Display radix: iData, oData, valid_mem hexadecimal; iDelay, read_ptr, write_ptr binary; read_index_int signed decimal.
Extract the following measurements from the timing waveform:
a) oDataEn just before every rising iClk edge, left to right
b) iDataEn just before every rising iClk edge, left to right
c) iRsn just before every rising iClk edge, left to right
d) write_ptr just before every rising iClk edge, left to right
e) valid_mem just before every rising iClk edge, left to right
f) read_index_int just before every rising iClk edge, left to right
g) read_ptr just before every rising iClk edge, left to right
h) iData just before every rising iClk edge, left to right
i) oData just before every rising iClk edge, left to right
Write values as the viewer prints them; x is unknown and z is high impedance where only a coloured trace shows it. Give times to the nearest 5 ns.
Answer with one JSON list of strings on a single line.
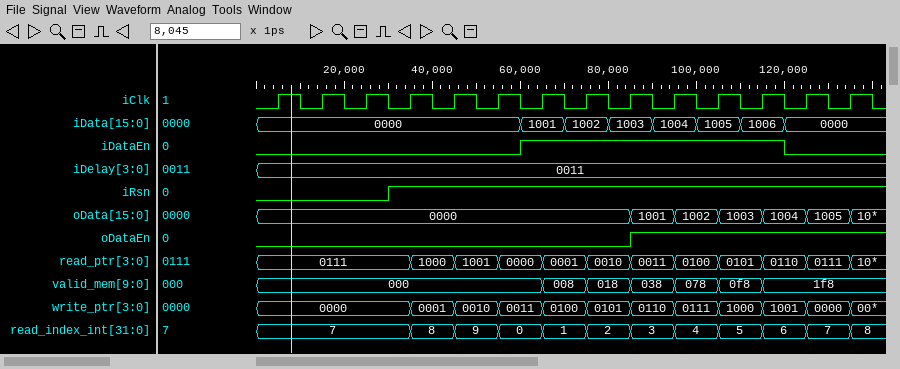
["0 0 0 0 0 0 0 0 0 1 1 1 1 1", "0 0 0 0 0 0 1 1 1 1 1 1 0 0", "0 0 0 1 1 1 1 1 1 1 1 1 1 1", "0000, 0000, 0000, 0000, 0001, 0010, 0011, 0100, 0101, 0110, 0111, 1000, 1001, 0000", "000, 000, 000, 000, 000, 000, 000, 008, 018, 038, 078, 0f8, 1f8, 1f8", "7, 7, 7, 7, 8, 9, 0, 1, 2, 3, 4, 5, 6, 7", "0111, 0111, 0111, 0111, 1000, 1001, 0000, 0001, 0010, 0011, 0100, 0101, 0110, 0111", "0000, 0000, 0000, 0000, 0000, 0000, 1001, 1002, 1003, 1004, 1005, 1006, 0000, 0000", "0000, 0000, 0000, 0000, 0000, 0000, 0000, 0000, 0000, 1001, 1002, 1003, 1004, 1005"]
